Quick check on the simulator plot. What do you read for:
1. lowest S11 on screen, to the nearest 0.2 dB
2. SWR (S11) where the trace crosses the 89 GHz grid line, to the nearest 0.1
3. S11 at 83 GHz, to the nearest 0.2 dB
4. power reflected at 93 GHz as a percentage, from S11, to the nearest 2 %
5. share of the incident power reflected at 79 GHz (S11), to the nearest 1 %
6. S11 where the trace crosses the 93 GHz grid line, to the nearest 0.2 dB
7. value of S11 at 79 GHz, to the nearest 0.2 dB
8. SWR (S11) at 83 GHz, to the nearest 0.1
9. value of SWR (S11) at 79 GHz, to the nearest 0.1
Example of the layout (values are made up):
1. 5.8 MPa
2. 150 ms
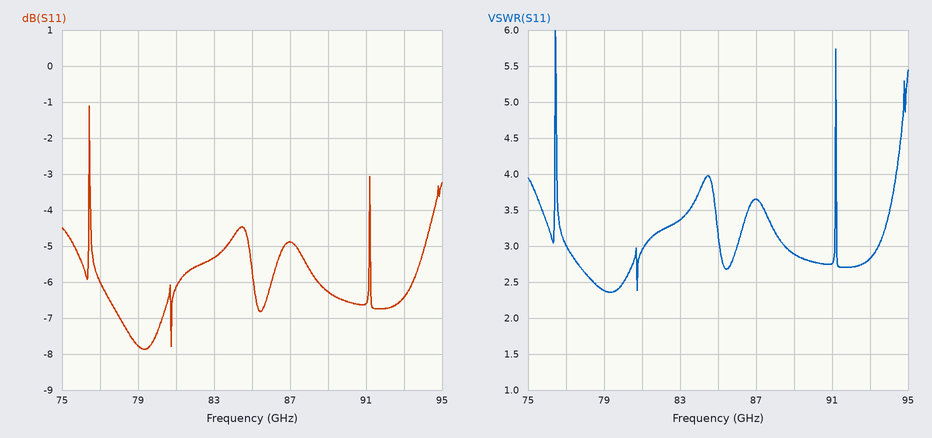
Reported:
1. -7.8 dB
2. 2.9
3. -5.4 dB
4. 22 %
5. 17 %
6. -6.4 dB
7. -7.8 dB
8. 3.4
9. 2.4
